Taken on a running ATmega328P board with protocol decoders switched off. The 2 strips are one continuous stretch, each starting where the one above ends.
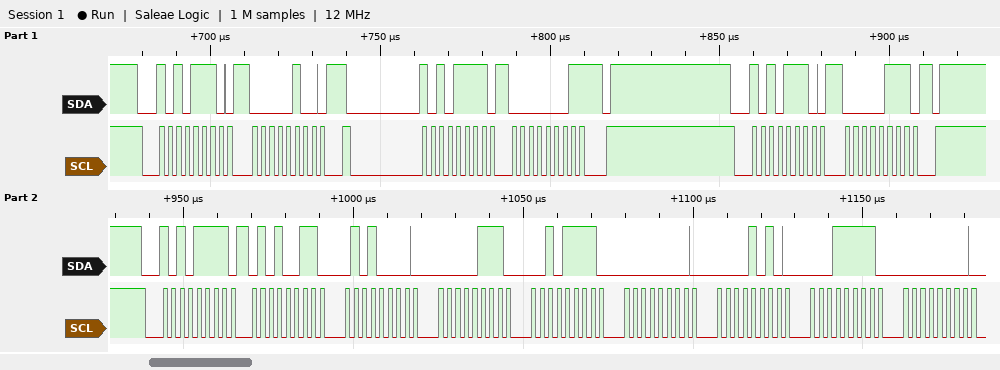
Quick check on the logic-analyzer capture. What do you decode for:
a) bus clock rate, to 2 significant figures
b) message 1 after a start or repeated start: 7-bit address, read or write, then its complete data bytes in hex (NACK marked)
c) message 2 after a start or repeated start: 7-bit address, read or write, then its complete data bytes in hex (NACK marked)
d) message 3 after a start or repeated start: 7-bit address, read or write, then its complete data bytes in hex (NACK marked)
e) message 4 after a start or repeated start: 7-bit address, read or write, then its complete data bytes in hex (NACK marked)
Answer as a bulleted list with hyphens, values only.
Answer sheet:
- 400 kHz
- 0x57 write: 04
- 0x57 read: 01 NACK
- 0x57 write: 07
- 0x57 read: 53 50 07 2F 00 0A 1F 00
